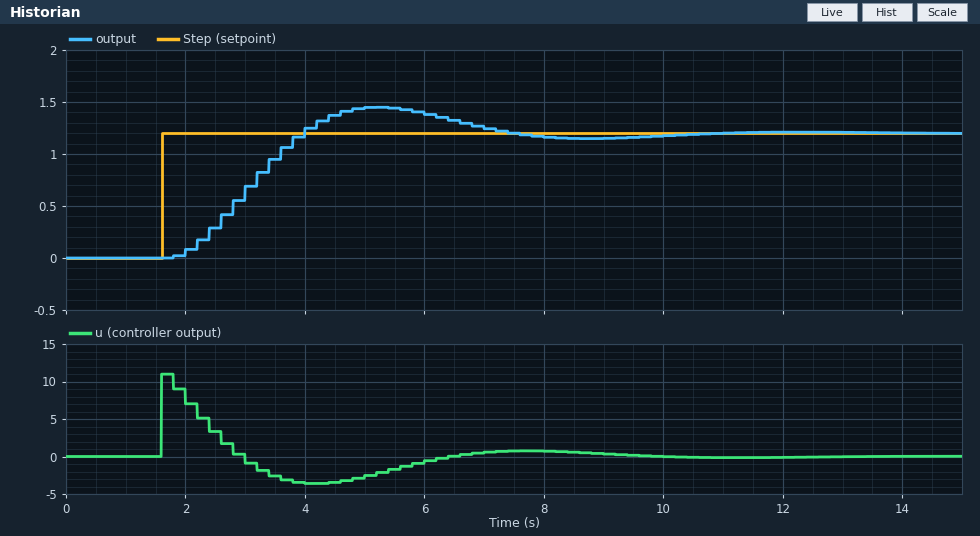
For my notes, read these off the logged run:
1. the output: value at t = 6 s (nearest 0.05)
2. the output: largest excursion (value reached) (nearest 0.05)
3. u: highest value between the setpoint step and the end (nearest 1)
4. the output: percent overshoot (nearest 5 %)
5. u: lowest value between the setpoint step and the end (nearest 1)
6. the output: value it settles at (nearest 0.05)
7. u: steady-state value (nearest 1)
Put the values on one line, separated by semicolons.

1.40; 1.45; 11; 20 %; -4; 1.20; 0
